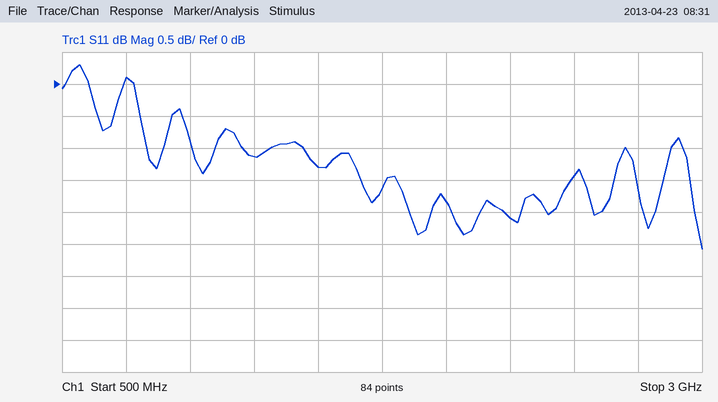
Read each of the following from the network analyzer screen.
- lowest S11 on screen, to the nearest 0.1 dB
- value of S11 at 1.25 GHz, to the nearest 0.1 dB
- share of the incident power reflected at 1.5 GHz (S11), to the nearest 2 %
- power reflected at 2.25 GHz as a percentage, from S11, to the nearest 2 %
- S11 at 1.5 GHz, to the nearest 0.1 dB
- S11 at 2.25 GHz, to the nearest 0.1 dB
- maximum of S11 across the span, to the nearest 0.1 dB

-2.6 dB
-1.1 dB
74 %
62 %
-1.3 dB
-2.1 dB
0.3 dB
